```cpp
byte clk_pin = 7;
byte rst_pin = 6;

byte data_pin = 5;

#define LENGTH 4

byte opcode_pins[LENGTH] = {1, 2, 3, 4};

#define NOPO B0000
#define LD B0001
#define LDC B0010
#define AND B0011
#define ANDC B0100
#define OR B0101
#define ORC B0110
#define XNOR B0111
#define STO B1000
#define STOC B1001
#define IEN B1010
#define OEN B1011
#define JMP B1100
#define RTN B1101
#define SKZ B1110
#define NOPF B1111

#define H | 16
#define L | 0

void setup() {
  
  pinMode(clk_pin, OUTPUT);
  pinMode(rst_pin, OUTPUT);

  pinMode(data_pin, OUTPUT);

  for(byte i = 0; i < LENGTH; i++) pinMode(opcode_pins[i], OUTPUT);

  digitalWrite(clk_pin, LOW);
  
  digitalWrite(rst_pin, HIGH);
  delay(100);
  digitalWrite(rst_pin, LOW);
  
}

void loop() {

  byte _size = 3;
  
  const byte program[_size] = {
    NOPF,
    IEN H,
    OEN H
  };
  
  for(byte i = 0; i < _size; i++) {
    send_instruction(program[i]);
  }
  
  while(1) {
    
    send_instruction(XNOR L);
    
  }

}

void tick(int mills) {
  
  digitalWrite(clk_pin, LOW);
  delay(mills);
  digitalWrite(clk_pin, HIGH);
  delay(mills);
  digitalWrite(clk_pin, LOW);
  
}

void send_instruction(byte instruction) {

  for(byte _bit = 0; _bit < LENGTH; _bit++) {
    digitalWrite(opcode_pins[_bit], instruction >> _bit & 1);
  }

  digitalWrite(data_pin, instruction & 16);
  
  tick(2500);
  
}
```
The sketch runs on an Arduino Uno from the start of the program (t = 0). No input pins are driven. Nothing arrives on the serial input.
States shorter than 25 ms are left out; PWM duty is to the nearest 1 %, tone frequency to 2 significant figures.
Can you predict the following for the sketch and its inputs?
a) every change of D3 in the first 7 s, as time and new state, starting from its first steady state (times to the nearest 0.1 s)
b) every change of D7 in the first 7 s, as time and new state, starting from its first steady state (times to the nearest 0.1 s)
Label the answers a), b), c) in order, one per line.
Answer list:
a) 0 s low; 0.1 s high; 5.1 s low
b) 0 s low; 2.6 s high; 5.1 s low
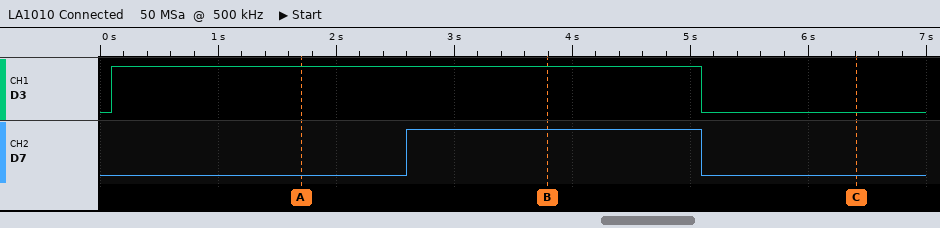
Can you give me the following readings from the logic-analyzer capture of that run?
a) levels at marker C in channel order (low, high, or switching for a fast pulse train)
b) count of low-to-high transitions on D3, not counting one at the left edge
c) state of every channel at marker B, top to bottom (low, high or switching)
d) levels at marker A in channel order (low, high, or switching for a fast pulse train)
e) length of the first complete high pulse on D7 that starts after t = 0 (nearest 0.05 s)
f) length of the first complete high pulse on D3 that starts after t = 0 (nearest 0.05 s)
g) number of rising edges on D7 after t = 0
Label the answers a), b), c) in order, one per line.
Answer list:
a) D3 low, D7 low
b) 1
c) D3 high, D7 high
d) D3 high, D7 low
e) 2.50 s
f) 5.00 s
g) 1
